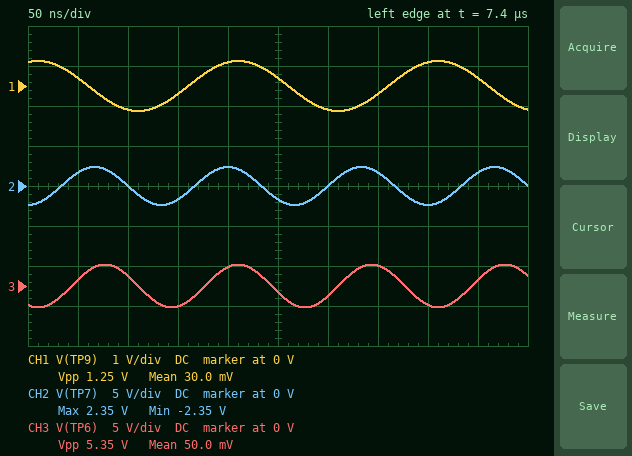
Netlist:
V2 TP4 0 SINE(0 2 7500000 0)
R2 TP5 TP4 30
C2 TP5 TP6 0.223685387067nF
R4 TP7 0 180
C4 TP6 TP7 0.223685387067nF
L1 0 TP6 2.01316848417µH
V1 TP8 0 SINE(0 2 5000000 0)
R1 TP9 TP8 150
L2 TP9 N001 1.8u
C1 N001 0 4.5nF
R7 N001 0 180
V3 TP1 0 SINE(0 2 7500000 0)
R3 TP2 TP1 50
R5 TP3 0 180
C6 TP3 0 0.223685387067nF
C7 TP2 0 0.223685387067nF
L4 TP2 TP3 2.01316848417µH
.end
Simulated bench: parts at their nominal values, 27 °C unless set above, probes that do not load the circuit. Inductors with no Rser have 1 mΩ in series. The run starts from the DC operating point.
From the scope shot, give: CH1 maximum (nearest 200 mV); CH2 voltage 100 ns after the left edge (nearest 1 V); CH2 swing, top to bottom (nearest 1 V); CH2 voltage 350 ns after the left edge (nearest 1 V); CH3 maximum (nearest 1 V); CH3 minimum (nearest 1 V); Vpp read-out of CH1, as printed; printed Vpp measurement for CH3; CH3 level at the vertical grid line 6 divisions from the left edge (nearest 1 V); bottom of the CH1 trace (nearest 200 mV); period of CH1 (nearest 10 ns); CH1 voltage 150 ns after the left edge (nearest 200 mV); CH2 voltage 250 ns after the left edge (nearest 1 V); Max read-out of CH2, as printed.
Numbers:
600 mV
0 V
5 V
2 V
3 V
-3 V
1.25 V
5.35 V
-1 V
-600 mV
200 ns
-200 mV
-2 V
2.35 V
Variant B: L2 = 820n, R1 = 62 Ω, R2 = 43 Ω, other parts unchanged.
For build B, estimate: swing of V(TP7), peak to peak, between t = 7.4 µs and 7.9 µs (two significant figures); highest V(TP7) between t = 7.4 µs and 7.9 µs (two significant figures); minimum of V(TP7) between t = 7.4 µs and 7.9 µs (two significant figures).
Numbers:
4.1 V
2.0 V
-2.0 V
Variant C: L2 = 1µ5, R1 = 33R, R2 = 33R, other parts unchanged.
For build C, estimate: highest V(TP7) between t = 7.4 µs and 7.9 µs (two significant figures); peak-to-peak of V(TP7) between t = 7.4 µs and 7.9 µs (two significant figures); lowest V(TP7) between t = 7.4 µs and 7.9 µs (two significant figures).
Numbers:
2.3 V
4.6 V
-2.3 V
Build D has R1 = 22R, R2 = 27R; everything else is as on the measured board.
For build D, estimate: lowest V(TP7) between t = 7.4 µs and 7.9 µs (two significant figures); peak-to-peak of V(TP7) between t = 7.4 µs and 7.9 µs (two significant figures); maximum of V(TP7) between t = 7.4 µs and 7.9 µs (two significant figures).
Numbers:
-2.5 V
4.9 V
2.5 V
